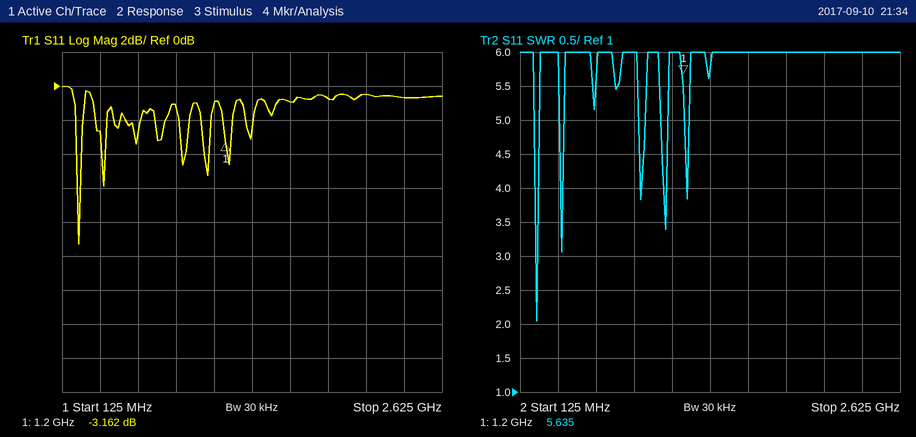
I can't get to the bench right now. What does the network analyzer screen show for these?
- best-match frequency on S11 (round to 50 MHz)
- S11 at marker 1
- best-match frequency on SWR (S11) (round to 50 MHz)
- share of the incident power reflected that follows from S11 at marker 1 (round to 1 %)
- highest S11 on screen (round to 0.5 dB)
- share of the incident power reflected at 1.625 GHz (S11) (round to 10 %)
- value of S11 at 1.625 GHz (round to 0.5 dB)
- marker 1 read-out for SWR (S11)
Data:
250 MHz
-3.162 dB
250 MHz
48 %
0.0 dB
80 %
-1.0 dB
5.635
